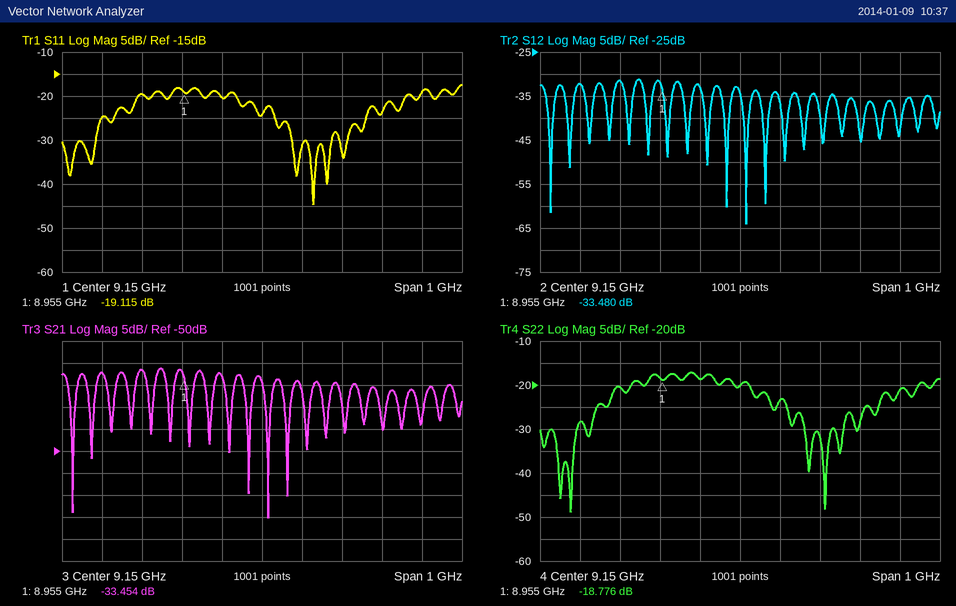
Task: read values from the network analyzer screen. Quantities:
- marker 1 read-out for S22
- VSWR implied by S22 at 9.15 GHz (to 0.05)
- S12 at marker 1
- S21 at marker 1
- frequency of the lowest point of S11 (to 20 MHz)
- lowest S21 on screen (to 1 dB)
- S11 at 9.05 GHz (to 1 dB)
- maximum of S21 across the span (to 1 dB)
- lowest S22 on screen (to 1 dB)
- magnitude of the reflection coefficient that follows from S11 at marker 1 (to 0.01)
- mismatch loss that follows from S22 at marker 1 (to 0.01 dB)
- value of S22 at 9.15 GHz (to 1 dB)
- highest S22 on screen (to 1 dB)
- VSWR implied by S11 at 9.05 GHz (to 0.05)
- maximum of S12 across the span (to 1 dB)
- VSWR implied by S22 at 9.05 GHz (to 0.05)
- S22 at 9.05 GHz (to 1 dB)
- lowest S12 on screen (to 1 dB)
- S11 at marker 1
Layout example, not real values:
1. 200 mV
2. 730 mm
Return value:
1. -18.776 dB
2. 1.20
3. -33.480 dB
4. -33.454 dB
5. 9.28 GHz
6. -65 dB
7. -20 dB
8. -31 dB
9. -49 dB
10. 0.11
11. 0.06 dB
12. -20 dB
13. -17 dB
14. 1.20
15. -31 dB
16. 1.25
17. -19 dB
18. -64 dB
19. -19.115 dB
